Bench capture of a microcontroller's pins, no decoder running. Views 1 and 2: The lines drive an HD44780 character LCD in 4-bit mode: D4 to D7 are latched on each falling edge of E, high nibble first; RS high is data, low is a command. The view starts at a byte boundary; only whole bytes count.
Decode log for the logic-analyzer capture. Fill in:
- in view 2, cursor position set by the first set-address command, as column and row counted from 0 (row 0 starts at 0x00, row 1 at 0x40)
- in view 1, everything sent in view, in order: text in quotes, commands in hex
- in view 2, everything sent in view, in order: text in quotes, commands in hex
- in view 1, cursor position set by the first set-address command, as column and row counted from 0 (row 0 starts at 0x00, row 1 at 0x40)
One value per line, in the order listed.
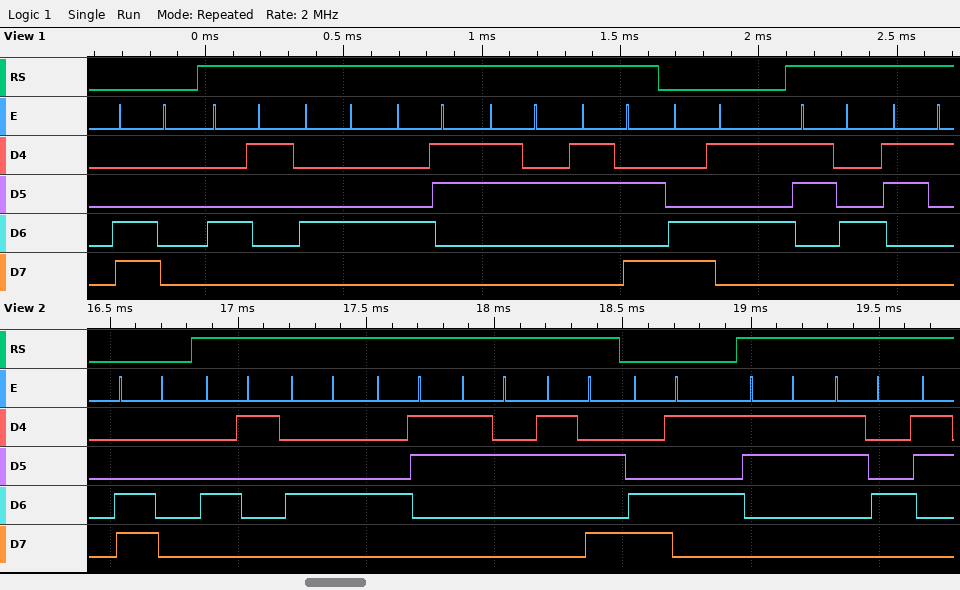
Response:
column 0, row 1
0xC0 "ADC2:" 0xC5 "41"
0xC0 "ADC2:" 0xC5 "34"
column 0, row 1
